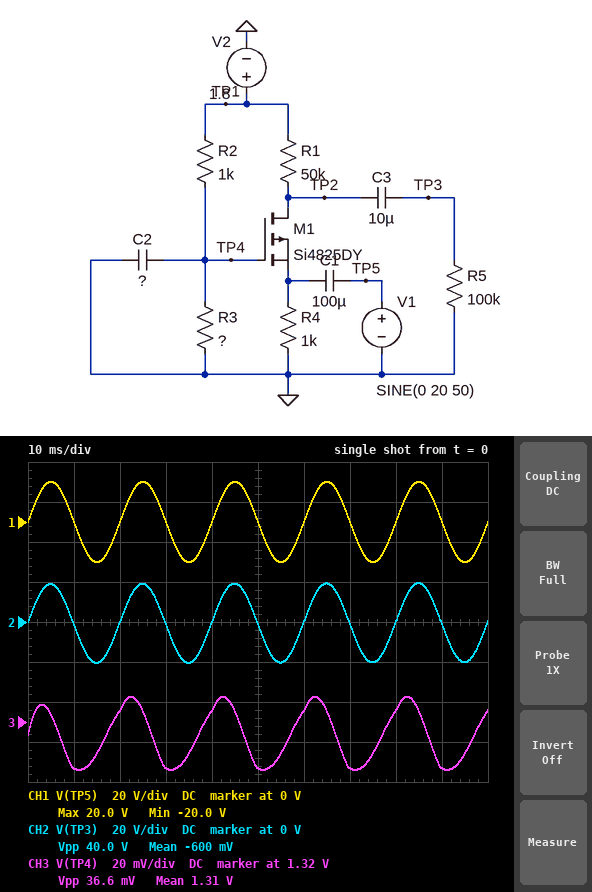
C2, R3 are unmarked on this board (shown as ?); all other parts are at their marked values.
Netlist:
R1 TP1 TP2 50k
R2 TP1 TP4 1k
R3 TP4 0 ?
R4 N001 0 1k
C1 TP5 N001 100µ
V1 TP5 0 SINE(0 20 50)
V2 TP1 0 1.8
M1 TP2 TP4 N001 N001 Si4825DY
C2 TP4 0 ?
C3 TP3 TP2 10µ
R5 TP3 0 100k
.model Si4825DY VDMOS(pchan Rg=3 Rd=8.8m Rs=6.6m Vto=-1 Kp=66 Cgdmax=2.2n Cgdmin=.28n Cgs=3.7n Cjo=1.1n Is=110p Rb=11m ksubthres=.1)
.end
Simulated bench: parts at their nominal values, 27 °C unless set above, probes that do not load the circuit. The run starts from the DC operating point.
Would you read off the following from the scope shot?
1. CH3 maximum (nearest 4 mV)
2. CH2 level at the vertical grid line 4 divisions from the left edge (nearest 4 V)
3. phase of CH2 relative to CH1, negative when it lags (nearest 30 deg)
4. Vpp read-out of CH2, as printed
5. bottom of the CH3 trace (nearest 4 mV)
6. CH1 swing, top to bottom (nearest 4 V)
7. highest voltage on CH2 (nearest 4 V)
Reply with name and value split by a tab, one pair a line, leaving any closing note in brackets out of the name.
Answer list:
CH3 maximum	1.332 V
CH2 level at the vertical grid line 4 divisions from the left edge	0 V
phase of CH2 relative to CH1, negative when it lags	0 deg
Vpp read-out of CH2, as printed	40.0 V
bottom of the CH3 trace	1.296 V
CH1 swing, top to bottom	40 V
highest voltage on CH2	20 V
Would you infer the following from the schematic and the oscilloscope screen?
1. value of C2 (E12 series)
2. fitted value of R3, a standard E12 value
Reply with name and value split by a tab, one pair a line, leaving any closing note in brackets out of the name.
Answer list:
value of C2	3.3 µF
fitted value of R3, a standard E12 value	2.7 kΩ
